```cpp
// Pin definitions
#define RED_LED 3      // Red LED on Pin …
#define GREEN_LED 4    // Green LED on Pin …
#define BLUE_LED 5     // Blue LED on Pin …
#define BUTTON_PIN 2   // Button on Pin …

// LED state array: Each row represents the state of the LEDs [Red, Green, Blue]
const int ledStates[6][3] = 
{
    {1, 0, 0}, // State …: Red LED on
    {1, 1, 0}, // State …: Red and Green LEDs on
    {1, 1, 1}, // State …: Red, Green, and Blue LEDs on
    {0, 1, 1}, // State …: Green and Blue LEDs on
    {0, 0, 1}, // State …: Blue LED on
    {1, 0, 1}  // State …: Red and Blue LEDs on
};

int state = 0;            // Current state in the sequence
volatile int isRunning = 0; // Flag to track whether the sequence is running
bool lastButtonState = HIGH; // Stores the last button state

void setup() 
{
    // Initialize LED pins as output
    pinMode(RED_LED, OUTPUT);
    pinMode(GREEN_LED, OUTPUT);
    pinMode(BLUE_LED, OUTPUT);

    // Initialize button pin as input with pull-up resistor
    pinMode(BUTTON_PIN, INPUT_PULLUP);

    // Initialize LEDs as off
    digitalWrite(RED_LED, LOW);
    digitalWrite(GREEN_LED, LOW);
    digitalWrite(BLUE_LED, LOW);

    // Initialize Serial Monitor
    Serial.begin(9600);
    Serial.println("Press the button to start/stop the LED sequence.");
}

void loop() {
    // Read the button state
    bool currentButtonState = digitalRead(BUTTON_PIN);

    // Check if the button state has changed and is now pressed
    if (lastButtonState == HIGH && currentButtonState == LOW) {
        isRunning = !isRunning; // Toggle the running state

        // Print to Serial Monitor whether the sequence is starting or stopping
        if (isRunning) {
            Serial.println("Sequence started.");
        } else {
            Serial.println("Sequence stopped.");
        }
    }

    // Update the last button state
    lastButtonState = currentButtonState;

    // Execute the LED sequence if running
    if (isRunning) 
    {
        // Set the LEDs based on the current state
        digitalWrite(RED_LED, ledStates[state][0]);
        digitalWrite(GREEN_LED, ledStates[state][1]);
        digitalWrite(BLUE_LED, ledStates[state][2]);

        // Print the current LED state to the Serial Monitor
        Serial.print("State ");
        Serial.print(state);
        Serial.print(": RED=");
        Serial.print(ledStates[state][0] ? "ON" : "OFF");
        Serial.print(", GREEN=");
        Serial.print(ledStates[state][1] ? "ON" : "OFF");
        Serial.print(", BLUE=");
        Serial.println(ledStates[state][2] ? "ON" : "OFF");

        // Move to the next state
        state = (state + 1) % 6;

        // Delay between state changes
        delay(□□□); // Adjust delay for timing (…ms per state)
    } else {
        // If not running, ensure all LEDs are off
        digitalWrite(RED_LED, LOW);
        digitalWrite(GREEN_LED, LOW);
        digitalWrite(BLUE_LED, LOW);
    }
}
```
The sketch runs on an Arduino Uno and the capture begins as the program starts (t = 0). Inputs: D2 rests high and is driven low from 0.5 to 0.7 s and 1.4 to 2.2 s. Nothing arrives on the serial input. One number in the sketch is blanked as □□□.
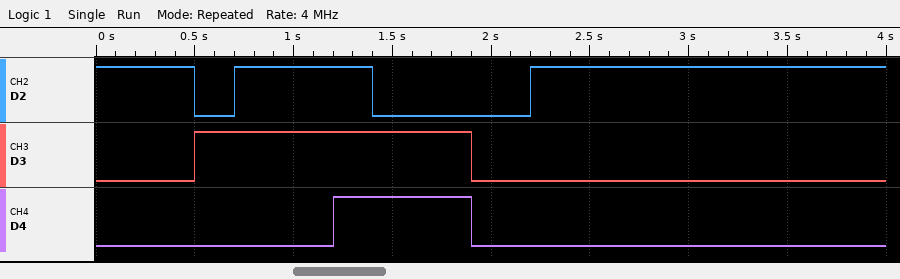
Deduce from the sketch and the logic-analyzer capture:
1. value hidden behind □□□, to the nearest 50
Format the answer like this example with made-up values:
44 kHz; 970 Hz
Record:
700
